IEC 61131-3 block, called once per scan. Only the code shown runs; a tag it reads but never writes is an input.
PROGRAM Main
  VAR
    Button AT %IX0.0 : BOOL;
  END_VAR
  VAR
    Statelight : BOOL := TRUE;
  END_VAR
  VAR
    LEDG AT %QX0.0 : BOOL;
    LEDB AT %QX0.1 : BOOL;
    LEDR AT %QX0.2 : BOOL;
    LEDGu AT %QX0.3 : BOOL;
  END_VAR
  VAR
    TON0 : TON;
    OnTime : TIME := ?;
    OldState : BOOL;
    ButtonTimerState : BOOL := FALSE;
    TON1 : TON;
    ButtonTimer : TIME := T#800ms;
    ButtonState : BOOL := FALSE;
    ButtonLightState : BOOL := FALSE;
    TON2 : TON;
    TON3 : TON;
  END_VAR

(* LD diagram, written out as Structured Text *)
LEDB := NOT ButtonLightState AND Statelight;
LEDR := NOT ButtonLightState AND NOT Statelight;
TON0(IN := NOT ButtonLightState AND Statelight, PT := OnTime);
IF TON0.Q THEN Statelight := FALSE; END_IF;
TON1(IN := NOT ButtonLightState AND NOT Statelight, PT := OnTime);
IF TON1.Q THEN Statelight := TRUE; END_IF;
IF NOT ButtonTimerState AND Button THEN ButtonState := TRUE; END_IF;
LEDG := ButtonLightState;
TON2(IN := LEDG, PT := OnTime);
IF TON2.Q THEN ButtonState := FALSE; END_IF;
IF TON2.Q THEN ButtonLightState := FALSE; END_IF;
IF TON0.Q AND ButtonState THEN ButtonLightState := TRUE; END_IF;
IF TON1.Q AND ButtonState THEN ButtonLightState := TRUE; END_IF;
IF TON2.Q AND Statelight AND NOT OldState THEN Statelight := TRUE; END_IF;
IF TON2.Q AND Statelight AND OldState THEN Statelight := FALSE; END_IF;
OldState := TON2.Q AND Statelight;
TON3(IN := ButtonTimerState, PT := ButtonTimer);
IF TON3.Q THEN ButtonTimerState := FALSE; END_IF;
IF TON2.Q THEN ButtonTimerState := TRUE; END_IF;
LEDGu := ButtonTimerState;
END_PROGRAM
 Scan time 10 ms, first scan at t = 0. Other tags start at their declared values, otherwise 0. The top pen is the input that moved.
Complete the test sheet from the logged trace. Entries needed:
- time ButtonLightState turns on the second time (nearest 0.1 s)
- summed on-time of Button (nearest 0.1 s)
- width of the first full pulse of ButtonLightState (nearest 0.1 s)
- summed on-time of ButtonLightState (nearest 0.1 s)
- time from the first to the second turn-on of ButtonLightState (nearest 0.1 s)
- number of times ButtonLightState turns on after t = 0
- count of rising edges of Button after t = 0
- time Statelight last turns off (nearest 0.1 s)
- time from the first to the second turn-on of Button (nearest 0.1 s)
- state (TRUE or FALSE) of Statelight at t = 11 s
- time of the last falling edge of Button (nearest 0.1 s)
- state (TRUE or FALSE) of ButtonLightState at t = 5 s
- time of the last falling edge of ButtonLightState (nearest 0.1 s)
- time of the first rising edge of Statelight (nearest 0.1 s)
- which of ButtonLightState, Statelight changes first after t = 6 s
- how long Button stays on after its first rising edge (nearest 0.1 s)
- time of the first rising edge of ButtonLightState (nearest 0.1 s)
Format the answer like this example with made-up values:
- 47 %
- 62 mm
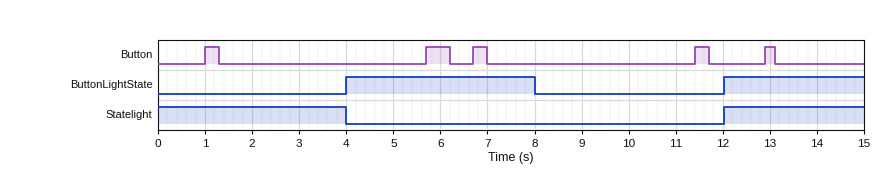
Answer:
- 12.0 s
- 1.6 s
- 4.0 s
- 7.0 s
- 8.0 s
- 2
- 5
- 4.0 s
- 4.7 s
- FALSE
- 13.1 s
- TRUE
- 8.0 s
- 12.0 s
- ButtonLightState
- 0.3 s
- 4.0 s
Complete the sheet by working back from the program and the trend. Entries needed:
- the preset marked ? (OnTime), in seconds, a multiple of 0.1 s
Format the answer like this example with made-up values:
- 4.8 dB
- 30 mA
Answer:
- 4.0 s
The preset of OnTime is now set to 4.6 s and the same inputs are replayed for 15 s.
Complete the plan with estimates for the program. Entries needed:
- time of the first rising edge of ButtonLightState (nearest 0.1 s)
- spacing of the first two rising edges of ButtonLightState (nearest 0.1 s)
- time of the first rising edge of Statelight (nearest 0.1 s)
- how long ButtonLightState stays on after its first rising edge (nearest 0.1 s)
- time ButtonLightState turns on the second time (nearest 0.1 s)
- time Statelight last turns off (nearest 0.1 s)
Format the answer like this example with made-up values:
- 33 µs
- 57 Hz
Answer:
- 4.6 s
- 9.2 s
- 13.8 s
- 4.6 s
- 13.8 s
- 4.6 s
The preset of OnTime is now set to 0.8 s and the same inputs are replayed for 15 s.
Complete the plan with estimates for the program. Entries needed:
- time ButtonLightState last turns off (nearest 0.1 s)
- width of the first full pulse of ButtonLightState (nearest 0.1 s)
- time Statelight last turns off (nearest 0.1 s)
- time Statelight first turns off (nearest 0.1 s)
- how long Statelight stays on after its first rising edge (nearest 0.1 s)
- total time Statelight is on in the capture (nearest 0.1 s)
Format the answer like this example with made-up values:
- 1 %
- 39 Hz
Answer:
- 12.9 s
- 0.8 s
- 14.5 s
- 0.8 s
- 1.6 s
- 7.3 s
